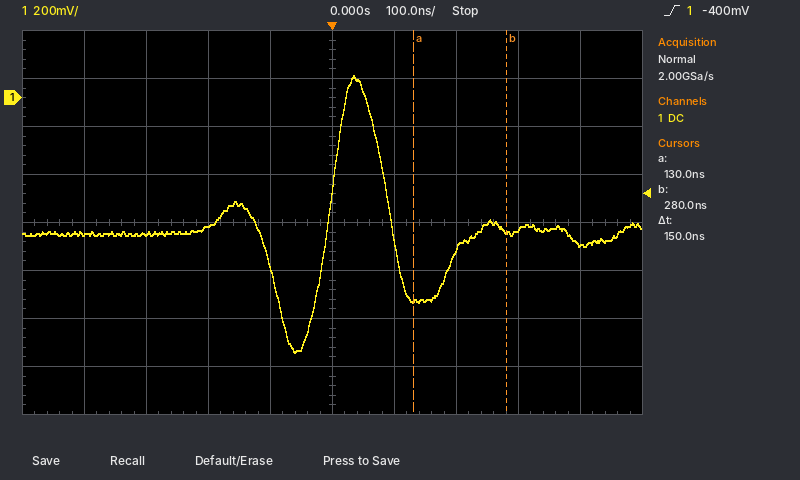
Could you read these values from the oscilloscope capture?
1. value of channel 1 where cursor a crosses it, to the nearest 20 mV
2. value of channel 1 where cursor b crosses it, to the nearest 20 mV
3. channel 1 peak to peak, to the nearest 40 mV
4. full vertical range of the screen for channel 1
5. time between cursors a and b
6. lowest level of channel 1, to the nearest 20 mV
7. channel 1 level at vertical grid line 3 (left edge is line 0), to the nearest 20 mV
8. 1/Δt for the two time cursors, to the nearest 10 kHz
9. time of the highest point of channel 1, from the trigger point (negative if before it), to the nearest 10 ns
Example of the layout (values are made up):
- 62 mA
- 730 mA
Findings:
- -840 mV
- -560 mV
- 1.16 V
- 1.6 V
- 150 ns
- -1.06 V
- -540 mV
- 6.67 MHz
- +40 ns
